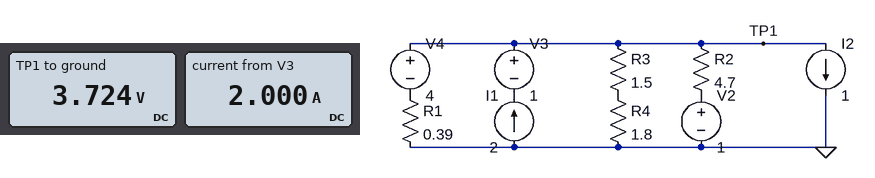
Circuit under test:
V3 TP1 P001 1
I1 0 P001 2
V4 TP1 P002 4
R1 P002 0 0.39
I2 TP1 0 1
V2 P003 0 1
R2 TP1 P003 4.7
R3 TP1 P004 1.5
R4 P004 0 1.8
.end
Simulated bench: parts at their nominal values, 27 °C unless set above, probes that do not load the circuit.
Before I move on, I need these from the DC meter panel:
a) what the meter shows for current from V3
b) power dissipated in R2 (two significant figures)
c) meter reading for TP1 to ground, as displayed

2.000 A
1.6 W
3.724 V
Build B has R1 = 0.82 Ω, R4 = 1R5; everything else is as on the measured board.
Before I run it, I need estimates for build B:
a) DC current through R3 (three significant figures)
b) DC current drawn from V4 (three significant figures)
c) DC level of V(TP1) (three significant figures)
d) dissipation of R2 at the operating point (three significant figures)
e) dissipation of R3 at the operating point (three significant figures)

1.15 A
671 mA
3.45 V
1.28 W
1.98 W
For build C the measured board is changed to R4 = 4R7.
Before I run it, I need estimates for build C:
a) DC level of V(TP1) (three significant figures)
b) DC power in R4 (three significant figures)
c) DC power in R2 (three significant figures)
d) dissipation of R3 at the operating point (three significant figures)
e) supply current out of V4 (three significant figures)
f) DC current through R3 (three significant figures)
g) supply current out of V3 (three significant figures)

3.90 V
1.86 W
1.79 W
595 mW
247 mA
630 mA
2.00 A
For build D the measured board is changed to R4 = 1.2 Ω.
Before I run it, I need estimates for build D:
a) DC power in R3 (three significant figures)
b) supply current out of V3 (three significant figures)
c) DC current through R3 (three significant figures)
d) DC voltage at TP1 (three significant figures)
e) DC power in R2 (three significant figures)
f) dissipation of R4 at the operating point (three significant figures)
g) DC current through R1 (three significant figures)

2.73 W
2.00 A
1.35 A
3.64 V
1.49 W
2.19 W
912 mA
